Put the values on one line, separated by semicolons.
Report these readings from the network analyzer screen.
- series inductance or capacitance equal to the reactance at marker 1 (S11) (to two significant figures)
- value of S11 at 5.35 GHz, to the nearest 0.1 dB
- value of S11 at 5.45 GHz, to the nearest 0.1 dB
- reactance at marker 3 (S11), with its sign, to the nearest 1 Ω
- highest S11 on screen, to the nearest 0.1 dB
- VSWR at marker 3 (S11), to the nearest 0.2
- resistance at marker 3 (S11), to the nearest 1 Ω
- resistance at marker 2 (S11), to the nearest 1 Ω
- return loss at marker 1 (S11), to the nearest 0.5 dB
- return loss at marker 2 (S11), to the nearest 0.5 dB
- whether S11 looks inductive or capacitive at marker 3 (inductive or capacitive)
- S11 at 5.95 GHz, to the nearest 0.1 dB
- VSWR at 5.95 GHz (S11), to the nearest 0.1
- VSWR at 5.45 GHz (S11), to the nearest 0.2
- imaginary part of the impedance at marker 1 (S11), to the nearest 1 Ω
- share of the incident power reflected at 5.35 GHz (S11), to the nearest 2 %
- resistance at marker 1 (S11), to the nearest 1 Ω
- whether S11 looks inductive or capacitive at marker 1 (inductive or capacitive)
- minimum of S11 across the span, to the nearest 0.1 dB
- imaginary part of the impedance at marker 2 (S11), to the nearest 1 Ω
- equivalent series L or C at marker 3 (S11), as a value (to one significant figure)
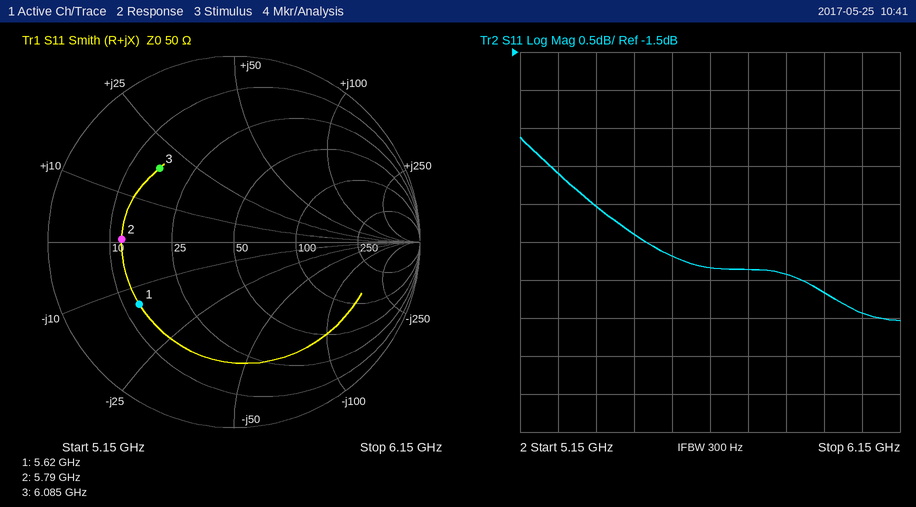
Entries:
2.0 pF; -3.5 dB; -3.9 dB; +19 Ω; -2.6 dB; 3.6; 16 Ω; 12 Ω; 4.5 dB; 4.5 dB; inductive; -4.7 dB; 3.8; 4.6; -14 Ω; 44 %; 13 Ω; capacitive; -5.0 dB; +1 Ω; 500 pH
